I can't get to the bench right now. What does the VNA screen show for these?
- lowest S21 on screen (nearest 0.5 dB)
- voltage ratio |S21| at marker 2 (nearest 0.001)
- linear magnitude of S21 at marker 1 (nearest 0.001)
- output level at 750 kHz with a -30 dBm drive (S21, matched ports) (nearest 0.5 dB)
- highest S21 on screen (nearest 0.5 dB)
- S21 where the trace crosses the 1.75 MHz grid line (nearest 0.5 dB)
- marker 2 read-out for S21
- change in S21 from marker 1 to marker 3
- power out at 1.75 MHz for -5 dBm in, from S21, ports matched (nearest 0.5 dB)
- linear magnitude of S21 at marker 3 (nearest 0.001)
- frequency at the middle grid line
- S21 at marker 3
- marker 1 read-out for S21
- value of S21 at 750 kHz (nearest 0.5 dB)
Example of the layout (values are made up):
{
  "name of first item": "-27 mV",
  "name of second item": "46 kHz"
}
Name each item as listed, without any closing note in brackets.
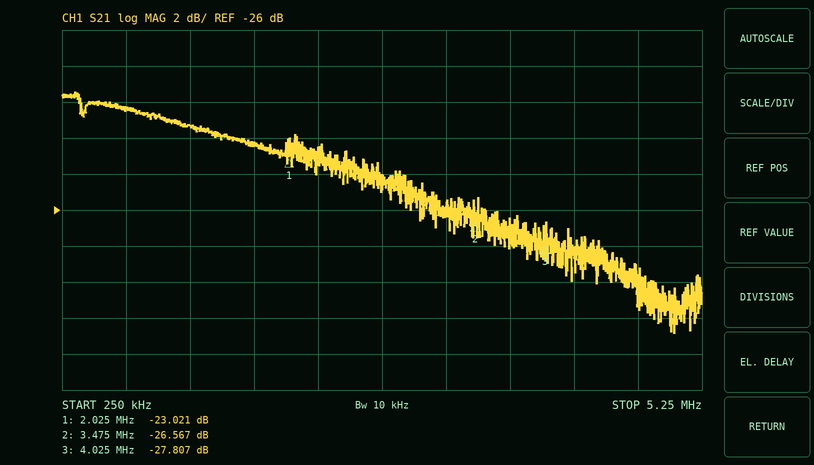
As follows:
{
  "lowest S21 on screen": "-33.0 dB",
  "voltage ratio |S21| at marker 2": "0.047",
  "linear magnitude of S21 at marker 1": "0.071",
  "output level at 750 kHz with a -30 dBm drive (S21, matched ports)": "-50.5 dBm",
  "highest S21 on screen": "-19.5 dB",
  "S21 where the trace crosses the 1.75 MHz grid line": "-22.5 dB",
  "marker 2 read-out for S21": "-26.567 dB",
  "change in S21 from marker 1 to marker 3": "-4.786 dB",
  "power out at 1.75 MHz for -5 dBm in, from S21, ports matched": "-27.5 dBm",
  "linear magnitude of S21 at marker 3": "0.041",
  "frequency at the middle grid line": "2.75 MHz",
  "S21 at marker 3": "-27.807 dB",
  "marker 1 read-out for S21": "-23.021 dB",
  "value of S21 at 750 kHz": "-20.5 dB"
}
